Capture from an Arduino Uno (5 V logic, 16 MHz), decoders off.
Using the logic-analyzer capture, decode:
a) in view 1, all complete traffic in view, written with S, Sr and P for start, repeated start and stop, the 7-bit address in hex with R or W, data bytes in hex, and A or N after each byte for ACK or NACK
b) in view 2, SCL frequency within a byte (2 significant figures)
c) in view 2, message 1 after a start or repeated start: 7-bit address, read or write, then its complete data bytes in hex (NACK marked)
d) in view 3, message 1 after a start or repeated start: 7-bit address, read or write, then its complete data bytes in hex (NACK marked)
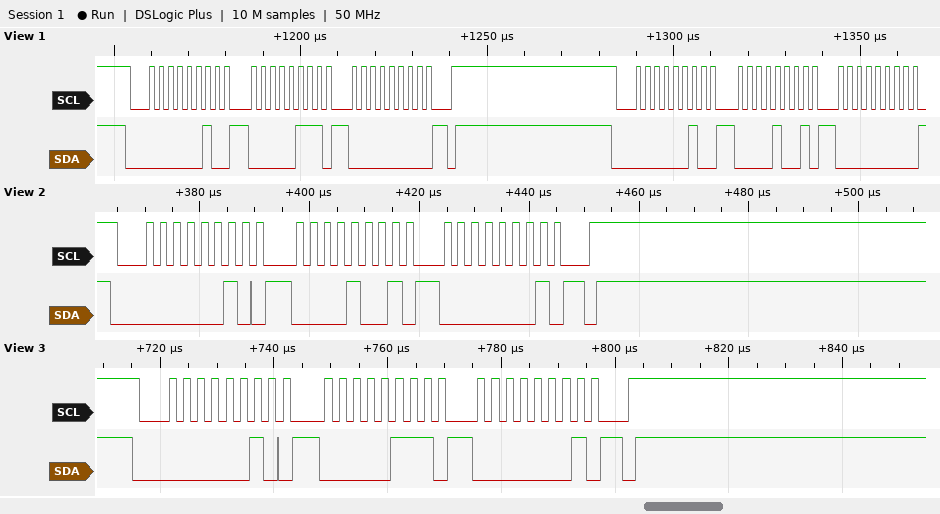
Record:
S 01W A 07 A 00 A P S 01W A 09 A 00 A
400 kHz
0x01 write: 09 01
0x01 write: 07 01
